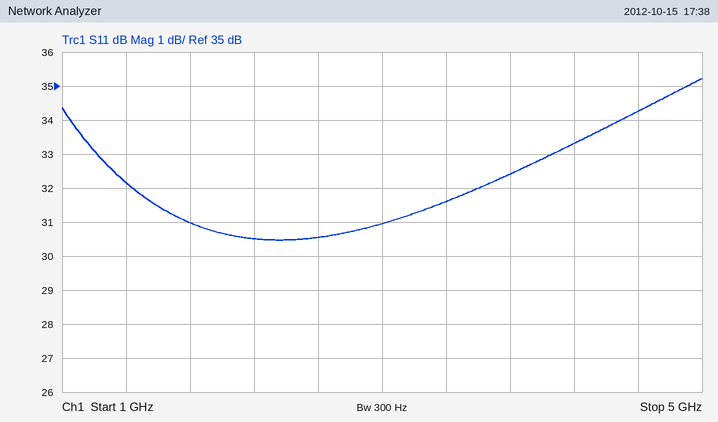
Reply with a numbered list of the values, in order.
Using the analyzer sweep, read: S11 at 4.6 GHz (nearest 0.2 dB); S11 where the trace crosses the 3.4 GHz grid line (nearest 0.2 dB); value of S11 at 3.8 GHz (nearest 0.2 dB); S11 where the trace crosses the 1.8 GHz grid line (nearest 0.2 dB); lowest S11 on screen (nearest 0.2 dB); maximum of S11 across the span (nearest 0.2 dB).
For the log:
1. 34.2 dB
2. 31.6 dB
3. 32.4 dB
4. 31.0 dB
5. 30.4 dB
6. 35.2 dB
